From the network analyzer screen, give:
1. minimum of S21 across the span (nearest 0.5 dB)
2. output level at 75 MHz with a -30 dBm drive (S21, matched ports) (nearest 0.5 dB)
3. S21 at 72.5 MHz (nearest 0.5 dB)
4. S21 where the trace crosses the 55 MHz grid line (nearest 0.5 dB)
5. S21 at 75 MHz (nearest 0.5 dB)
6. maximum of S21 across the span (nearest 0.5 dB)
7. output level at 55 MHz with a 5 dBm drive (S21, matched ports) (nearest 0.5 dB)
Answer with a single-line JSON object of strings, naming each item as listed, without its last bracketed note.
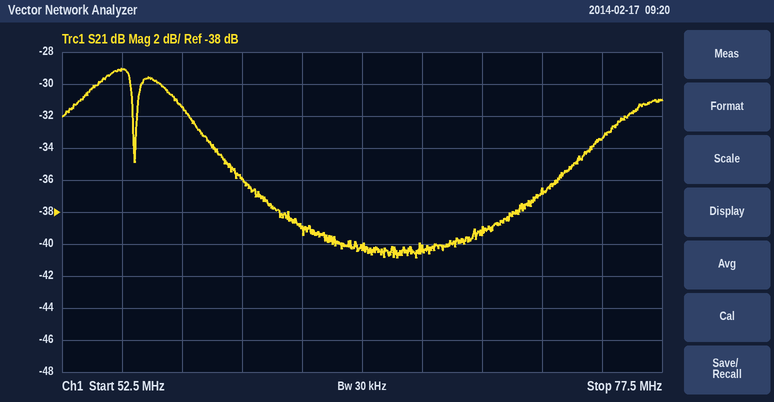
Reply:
{"minimum of S21 across the span": "-41.0 dB", "output level at 75 MHz with a -30 dBm drive (S21, matched ports)": "-63.5 dBm", "S21 at 72.5 MHz": "-36.5 dB", "S21 where the trace crosses the 55 MHz grid line": "-29.0 dB", "S21 at 75 MHz": "-33.5 dB", "maximum of S21 across the span": "-29.0 dB", "output level at 55 MHz with a 5 dBm drive (S21, matched ports)": "-24.0 dBm"}
